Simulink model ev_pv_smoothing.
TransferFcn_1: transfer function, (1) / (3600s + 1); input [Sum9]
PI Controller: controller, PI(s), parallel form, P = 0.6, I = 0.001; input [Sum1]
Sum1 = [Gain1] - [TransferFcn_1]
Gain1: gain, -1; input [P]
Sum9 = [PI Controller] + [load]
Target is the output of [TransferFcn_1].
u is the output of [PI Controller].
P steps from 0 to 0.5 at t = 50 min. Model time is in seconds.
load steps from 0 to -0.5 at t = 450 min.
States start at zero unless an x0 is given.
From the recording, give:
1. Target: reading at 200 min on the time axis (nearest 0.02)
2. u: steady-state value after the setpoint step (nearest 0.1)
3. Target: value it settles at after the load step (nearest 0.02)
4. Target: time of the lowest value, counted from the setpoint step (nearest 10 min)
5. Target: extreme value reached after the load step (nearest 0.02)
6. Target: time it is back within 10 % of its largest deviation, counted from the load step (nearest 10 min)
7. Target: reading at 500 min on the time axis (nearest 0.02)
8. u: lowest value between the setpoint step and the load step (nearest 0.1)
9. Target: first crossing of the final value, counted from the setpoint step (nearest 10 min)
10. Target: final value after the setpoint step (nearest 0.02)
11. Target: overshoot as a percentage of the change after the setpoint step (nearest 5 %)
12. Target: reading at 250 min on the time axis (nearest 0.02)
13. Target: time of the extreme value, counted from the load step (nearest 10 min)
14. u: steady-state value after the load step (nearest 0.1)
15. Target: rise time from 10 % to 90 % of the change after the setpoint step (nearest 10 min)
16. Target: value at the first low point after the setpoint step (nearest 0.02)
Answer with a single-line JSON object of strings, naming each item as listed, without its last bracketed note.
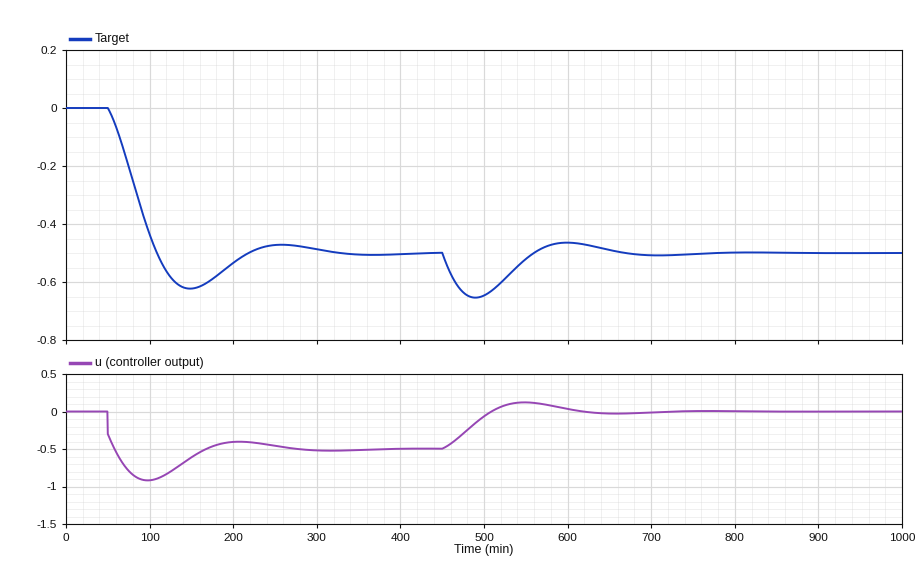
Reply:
{"Target: reading at 200 min on the time axis": "-0.54", "u: steady-state value after the setpoint step": "-0.5", "Target: value it settles at after the load step": "-0.50", "Target: time of the lowest value, counted from the setpoint step": "100 min", "Target: extreme value reached after the load step": "-0.66", "Target: time it is back within 10 % of its largest deviation, counted from the load step": "190 min", "Target: reading at 500 min on the time axis": "-0.64", "u: lowest value between the setpoint step and the load step": "-0.9", "Target: first crossing of the final value, counted from the setpoint step": "60 min", "Target: final value after the setpoint step": "-0.50", "Target: overshoot as a percentage of the change after the setpoint step": "25 %", "Target: reading at 250 min on the time axis": "-0.48", "Target: time of the extreme value, counted from the load step": "40 min", "u: steady-state value after the load step": "0.0", "Target: rise time from 10 % to 90 % of the change after the setpoint step": "40 min", "Target: value at the first low point after the setpoint step": "-0.62"}
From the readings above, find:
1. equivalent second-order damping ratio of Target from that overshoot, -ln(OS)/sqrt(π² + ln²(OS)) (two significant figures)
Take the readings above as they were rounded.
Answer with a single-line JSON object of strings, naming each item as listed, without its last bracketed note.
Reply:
{"equivalent second-order damping ratio of Target from that overshoot, -ln(OS)/sqrt(π² + ln²(OS))": "0.40"}
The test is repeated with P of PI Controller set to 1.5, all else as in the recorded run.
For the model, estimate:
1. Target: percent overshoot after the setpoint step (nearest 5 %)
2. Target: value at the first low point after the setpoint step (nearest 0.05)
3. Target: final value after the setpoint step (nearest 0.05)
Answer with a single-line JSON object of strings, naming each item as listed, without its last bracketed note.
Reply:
{"Target: percent overshoot after the setpoint step": "10 %", "Target: value at the first low point after the setpoint step": "-0.55", "Target: final value after the setpoint step": "-0.50"}
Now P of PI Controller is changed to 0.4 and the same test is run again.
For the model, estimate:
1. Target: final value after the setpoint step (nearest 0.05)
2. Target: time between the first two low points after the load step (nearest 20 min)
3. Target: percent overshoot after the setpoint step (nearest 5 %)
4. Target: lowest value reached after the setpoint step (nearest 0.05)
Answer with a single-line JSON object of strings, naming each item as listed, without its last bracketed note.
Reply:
{"Target: final value after the setpoint step": "-0.50", "Target: time between the first two low points after the load step": "220 min", "Target: percent overshoot after the setpoint step": "30 %", "Target: lowest value reached after the setpoint step": "-0.65"}
